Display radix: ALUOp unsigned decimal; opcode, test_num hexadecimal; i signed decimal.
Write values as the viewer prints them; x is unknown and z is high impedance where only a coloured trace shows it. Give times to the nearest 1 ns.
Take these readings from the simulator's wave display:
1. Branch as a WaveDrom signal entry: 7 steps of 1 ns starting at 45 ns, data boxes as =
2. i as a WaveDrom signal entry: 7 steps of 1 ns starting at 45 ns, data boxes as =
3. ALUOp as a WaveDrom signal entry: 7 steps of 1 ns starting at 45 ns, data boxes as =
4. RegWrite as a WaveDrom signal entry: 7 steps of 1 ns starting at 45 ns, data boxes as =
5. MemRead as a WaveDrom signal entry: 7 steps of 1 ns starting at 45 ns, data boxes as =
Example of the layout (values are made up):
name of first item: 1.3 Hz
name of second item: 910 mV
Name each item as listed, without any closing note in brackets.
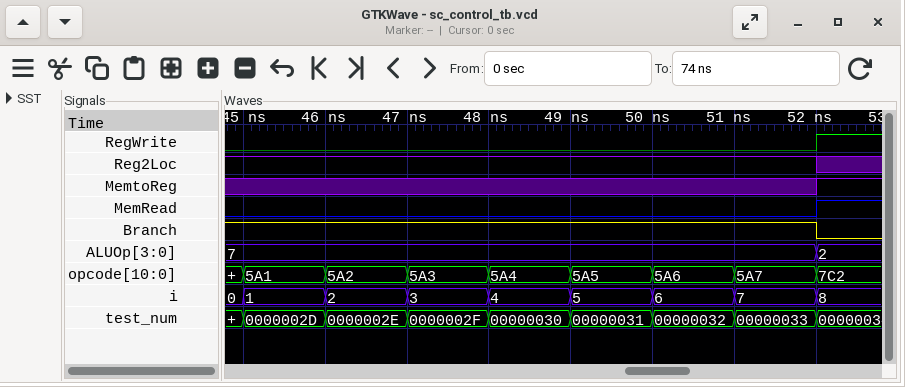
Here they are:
Branch as a WaveDrom signal entry: 7 steps of 1 ns starting at 45 ns, data boxes as =: {name: 'Branch', wave: '1......'}
i as a WaveDrom signal entry: 7 steps of 1 ns starting at 45 ns, data boxes as =: {name: 'i', wave: '=======', data: '1 2 3 4 5 6 7'}
ALUOp as a WaveDrom signal entry: 7 steps of 1 ns starting at 45 ns, data boxes as =: {name: 'ALUOp', wave: '=......', data: '7'}
RegWrite as a WaveDrom signal entry: 7 steps of 1 ns starting at 45 ns, data boxes as =: {name: 'RegWrite', wave: '0......'}
MemRead as a WaveDrom signal entry: 7 steps of 1 ns starting at 45 ns, data boxes as =: {name: 'MemRead', wave: '0......'}
